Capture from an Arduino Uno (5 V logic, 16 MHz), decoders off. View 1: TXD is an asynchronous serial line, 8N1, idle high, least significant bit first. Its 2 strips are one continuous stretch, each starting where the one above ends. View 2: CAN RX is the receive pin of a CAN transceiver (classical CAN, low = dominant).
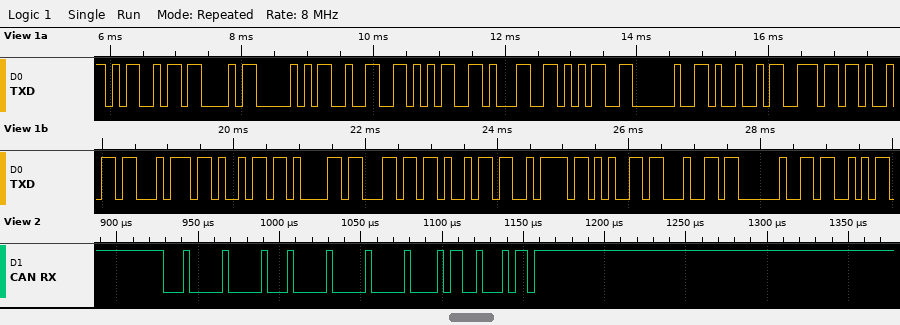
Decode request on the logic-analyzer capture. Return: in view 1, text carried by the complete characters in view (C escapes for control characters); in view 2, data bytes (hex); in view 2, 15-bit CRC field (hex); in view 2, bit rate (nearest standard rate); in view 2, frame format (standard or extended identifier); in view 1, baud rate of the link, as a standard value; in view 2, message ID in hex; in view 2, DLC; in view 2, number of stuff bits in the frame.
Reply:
"MCP2515 Initialized S"
00 00
0x1645
250 kbit/s
standard
9600 baud
0x100
2
5
